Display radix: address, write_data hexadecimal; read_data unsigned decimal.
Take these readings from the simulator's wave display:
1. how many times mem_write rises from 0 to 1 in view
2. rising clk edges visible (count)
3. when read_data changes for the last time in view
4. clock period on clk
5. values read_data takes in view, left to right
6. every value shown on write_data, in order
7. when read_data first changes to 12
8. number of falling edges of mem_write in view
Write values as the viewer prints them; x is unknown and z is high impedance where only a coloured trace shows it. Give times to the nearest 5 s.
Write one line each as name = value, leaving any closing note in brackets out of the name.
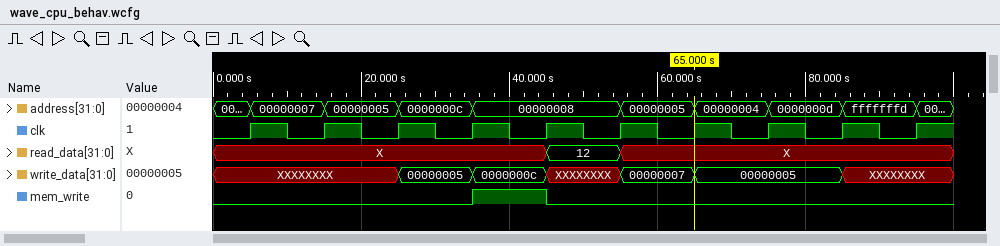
how many times mem_write rises from 0 to 1 in view = 1
rising clk edges visible = 10
when read_data changes for the last time in view = 55 s
clock period on clk = 10 s
values read_data takes in view, left to right = X, 12, X
every value shown on write_data, in order = XXXXXXXX, 00000005, 0000000c, XXXXXXXX, 00000007, 00000005, XXXXXXXX
when read_data first changes to 12 = 45 s
number of falling edges of mem_write in view = 1
